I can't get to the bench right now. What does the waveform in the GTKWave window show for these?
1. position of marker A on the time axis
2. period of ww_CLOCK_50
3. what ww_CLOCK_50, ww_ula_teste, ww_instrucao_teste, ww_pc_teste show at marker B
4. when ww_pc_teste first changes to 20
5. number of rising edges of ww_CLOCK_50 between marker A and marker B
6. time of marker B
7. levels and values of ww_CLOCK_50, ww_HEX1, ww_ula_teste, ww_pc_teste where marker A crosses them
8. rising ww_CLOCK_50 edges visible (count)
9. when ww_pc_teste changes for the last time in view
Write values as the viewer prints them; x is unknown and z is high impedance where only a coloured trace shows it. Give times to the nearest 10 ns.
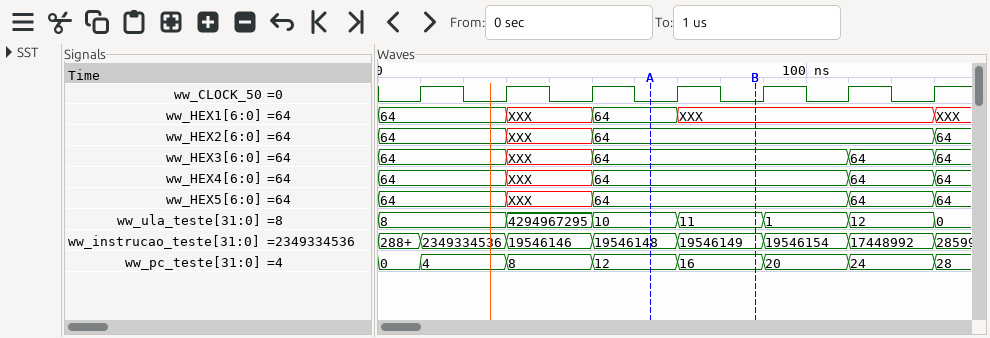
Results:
60 ns
20 ns
ww_CLOCK_50=0, ww_ula_teste=11, ww_instrucao_teste=19546149, ww_pc_teste=16
90 ns
1
90 ns
ww_CLOCK_50=0, ww_HEX1=64, ww_ula_teste=10, ww_pc_teste=12
7
130 ns
